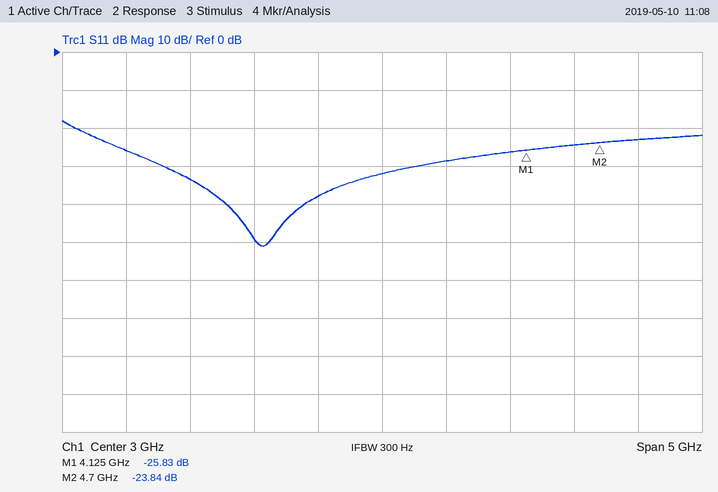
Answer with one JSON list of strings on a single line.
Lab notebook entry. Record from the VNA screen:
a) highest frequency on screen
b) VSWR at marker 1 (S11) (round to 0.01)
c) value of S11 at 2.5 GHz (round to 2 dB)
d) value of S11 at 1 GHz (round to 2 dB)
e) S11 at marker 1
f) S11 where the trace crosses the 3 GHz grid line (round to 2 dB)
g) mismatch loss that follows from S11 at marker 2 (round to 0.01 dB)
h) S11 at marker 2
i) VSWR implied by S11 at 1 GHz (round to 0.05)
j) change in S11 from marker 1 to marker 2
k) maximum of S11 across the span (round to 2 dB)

["5.5 GHz", "1.11", "-38 dB", "-26 dB", "-25.83 dB", "-32 dB", "0.02 dB", "-23.84 dB", "1.10", "1.99 dB", "-18 dB"]
